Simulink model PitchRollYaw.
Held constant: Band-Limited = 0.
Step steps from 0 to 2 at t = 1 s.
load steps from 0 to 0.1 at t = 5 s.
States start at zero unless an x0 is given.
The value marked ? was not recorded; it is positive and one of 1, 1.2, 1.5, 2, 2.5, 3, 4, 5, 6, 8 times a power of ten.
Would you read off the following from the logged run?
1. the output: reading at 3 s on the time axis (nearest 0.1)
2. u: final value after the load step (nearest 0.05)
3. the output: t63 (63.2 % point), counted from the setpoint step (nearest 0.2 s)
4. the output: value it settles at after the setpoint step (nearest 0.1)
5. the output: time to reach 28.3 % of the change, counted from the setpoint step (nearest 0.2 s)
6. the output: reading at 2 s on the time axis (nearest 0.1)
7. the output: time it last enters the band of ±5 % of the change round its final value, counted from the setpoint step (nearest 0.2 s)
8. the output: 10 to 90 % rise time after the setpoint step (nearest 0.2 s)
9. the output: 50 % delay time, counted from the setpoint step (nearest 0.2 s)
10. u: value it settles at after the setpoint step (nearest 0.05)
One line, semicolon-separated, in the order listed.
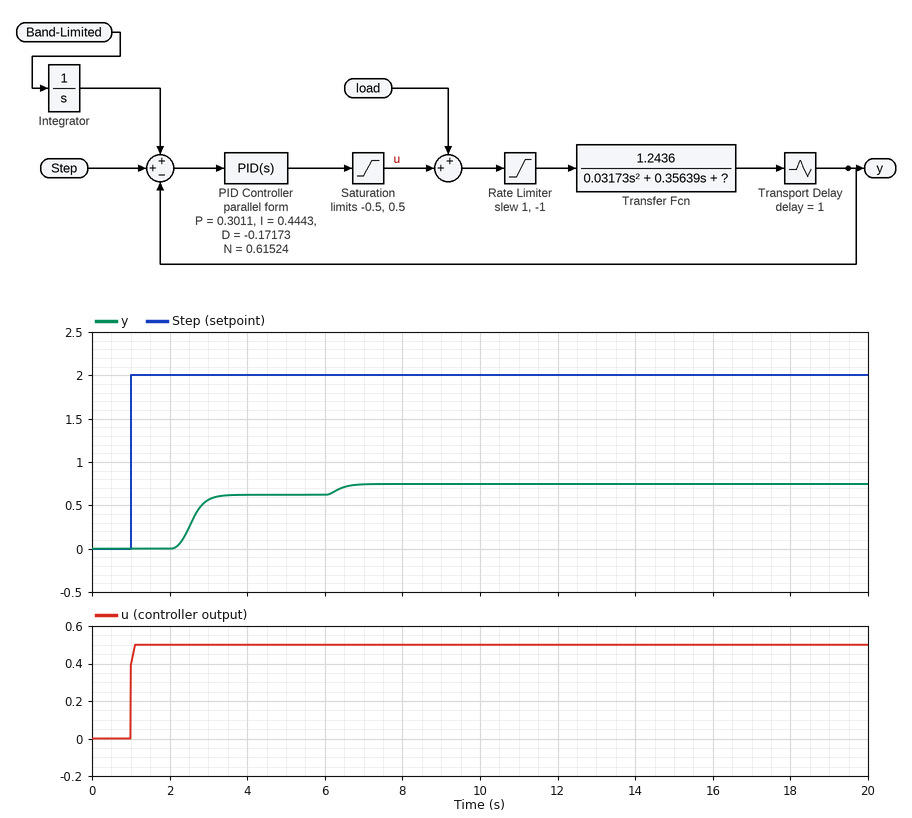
0.6; 0.50; 1.6 s; 0.6; 1.4 s; 0.0; 2.2 s; 0.8 s; 1.6 s; 0.50
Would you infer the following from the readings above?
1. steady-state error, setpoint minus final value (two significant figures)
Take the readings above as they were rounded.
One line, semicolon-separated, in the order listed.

1.4
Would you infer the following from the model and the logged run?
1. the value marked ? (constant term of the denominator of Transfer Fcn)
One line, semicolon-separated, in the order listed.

1
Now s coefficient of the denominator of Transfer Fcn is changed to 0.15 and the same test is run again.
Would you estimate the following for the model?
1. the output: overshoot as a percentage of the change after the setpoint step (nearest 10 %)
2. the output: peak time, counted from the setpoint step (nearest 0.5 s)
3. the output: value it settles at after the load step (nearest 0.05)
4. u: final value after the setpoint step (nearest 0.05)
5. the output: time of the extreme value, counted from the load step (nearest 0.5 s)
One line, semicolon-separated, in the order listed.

20 %; 2.0 s; 0.75; 0.50; 1.5 s
